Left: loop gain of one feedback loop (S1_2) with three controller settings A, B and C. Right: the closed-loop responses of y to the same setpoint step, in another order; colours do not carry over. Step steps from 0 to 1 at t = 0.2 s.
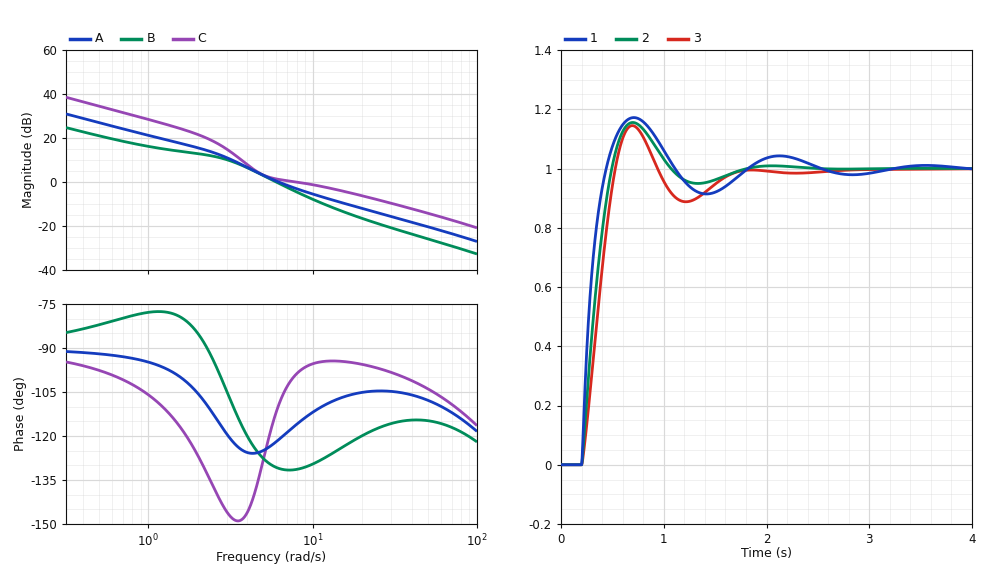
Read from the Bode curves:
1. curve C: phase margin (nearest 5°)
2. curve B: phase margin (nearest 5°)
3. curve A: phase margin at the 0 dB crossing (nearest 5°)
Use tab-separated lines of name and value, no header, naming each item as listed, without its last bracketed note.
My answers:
curve C: phase margin	80°
curve B: phase margin	50°
curve A: phase margin at the 0 dB crossing	60°
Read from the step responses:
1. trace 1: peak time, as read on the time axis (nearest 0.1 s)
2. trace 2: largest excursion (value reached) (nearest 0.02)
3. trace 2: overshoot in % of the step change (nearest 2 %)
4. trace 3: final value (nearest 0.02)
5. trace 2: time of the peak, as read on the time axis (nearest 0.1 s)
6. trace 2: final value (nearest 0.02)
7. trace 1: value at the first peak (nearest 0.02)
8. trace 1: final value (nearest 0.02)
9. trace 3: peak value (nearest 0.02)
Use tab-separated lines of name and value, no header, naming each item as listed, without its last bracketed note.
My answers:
trace 1: peak time, as read on the time axis	0.7 s
trace 2: largest excursion (value reached)	1.16
trace 2: overshoot in % of the step change	16 %
trace 3: final value	1.00
trace 2: time of the peak, as read on the time axis	0.7 s
trace 2: final value	1.00
trace 1: value at the first peak	1.18
trace 1: final value	1.00
trace 3: peak value	1.14
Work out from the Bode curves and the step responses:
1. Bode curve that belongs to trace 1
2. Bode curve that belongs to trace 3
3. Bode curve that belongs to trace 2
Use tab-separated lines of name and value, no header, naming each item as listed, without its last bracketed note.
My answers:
Bode curve that belongs to trace 1	C
Bode curve that belongs to trace 3	B
Bode curve that belongs to trace 2	A
